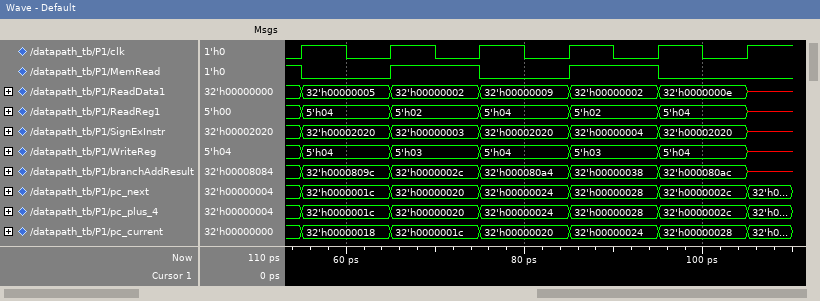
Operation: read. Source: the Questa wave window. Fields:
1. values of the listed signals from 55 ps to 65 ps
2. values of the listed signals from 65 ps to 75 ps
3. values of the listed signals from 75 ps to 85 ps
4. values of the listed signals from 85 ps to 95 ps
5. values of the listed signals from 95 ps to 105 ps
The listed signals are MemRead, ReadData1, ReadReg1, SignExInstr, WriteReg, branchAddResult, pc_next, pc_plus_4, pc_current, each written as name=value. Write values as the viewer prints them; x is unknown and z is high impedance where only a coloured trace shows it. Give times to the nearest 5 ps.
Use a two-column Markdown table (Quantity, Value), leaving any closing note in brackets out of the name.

| Quantity | Value |
|---|---|
| values of the listed signals from 55 ps to 65 ps | MemRead=0, ReadData1=32'h00000005, ReadReg1=5'h04, SignExInstr=32'h00002020, WriteReg=5'h04, branchAddResult=32'h0000809c, pc_next=32'h0000001c, pc_plus_4=32'h0000001c, pc_current=32'h00000018 |
| values of the listed signals from 65 ps to 75 ps | MemRead=1, ReadData1=32'h00000002, ReadReg1=5'h02, SignExInstr=32'h00000003, WriteReg=5'h03, branchAddResult=32'h0000002c, pc_next=32'h00000020, pc_plus_4=32'h00000020, pc_current=32'h0000001c |
| values of the listed signals from 75 ps to 85 ps | MemRead=0, ReadData1=32'h00000009, ReadReg1=5'h04, SignExInstr=32'h00002020, WriteReg=5'h04, branchAddResult=32'h000080a4, pc_next=32'h00000024, pc_plus_4=32'h00000024, pc_current=32'h00000020 |
| values of the listed signals from 85 ps to 95 ps | MemRead=1, ReadData1=32'h00000002, ReadReg1=5'h02, SignExInstr=32'h00000004, WriteReg=5'h03, branchAddResult=32'h00000038, pc_next=32'h00000028, pc_plus_4=32'h00000028, pc_current=32'h00000024 |
| values of the listed signals from 95 ps to 105 ps | MemRead=0, ReadData1=32'h0000000e, ReadReg1=5'h04, SignExInstr=32'h00002020, WriteReg=5'h04, branchAddResult=32'h000080ac, pc_next=32'h0000002c, pc_plus_4=32'h0000002c, pc_current=32'h00000028 |
